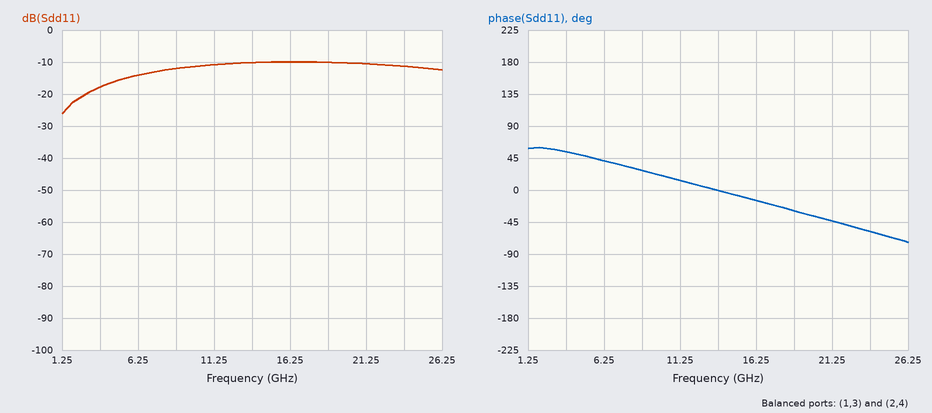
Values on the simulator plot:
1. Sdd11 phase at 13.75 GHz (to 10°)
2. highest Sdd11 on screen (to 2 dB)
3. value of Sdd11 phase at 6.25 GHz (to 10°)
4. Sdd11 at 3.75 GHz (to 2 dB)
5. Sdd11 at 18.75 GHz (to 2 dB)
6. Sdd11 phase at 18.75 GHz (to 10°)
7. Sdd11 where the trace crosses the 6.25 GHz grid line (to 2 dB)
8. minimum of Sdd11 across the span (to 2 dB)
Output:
0°
-10 dB
40°
-18 dB
-10 dB
-30°
-14 dB
-26 dB
